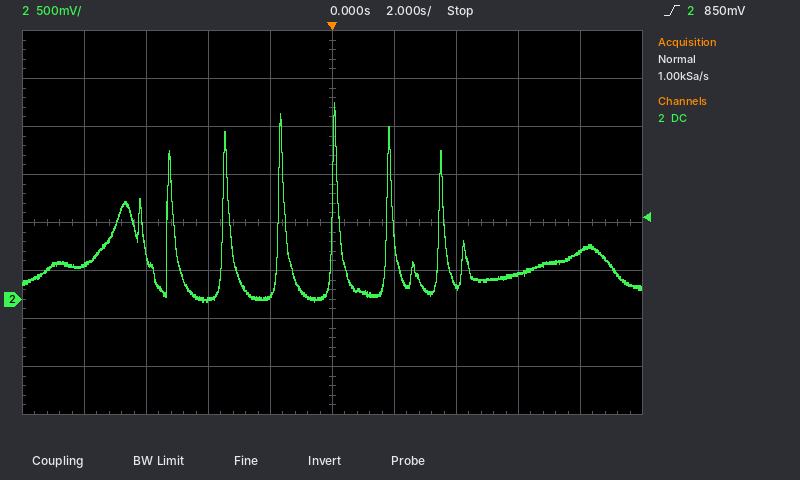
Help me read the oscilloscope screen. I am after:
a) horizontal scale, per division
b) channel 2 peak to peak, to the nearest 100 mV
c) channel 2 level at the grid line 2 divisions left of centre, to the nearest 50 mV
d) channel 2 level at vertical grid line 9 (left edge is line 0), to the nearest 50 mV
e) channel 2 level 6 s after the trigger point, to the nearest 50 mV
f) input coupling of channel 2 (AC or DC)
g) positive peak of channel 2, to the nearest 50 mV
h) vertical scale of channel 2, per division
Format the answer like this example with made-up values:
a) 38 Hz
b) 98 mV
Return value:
a) 2 s
b) 2.10 V
c) 0 mV
d) 500 mV
e) 250 mV
f) DC
g) 2.05 V
h) 500 mV
